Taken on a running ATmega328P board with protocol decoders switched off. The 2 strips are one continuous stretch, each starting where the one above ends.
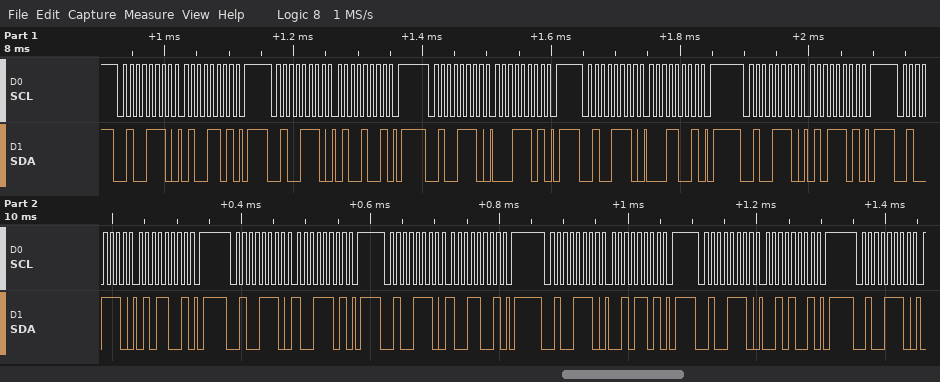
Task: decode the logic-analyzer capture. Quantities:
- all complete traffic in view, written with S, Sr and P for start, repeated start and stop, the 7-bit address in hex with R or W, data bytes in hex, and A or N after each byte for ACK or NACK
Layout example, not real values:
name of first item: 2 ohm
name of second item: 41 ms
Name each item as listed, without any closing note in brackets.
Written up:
all complete traffic in view, written with S, Sr and P for start, repeated start and stop, the 7-bit address in hex with R or W, data bytes in hex, and A or N after each byte for ACK or NACK: S 27W A 4D A P S 27W A 49 A P S 27W A 1D A P S 27W A 19 A P S 27W A 5D A P S 27W A 59 A P S 27W A 9D A P S 27W A 99 A P S 27W A 2D A P S 27W A 29 A P S 27W A
